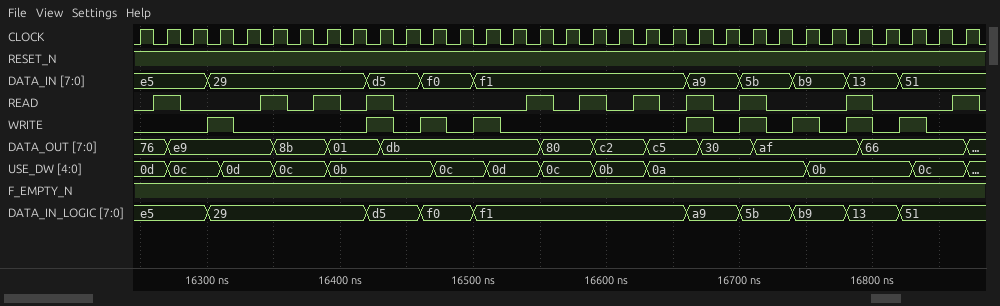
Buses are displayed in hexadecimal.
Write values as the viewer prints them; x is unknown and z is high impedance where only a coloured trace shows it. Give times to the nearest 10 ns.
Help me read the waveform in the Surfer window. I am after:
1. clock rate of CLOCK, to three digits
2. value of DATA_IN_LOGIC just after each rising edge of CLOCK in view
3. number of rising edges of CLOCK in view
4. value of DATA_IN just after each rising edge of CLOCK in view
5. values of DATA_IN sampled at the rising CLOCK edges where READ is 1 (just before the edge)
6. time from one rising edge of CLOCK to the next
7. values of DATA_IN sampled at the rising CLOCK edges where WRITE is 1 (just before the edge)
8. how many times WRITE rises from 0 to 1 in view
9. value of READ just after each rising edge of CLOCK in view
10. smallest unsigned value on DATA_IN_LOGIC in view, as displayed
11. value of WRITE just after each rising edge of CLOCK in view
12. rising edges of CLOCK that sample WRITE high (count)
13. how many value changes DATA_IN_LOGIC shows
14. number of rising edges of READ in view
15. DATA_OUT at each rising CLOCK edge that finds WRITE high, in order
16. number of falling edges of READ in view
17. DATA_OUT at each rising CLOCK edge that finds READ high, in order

50.0 MHz
e5, e5, e5, 29, 29, 29, 29, 29, 29, d5, d5, f0, f0, f1, f1, f1, f1, f1, f1, f1, f1, a9, a9, 5b, 5b, b9, b9, 13, 13, 51, 51, 51
32
e5, e5, e5, 29, 29, 29, 29, 29, 29, d5, d5, f0, f0, f1, f1, f1, f1, f1, f1, f1, f1, a9, a9, 5b, 5b, b9, b9, 13, 13, 51, 51, 51
e5, 29, 29, d5, f1, f1, f1, a9, 5b, 13, 51
20 ns
29, d5, f0, f1, a9, 5b, b9, 13, 51
9
0 1 0 0 0 1 0 1 0 1 0 0 0 0 0 1 0 1 0 1 0 1 0 1 0 0 0 1 0 0 0 1
13
0 0 0 1 0 0 0 0 0 1 0 1 0 1 0 0 0 0 0 0 0 1 0 1 0 1 0 1 0 1 0 0
9
9
11
e9, 01, db, db, c5, 30, af, af, 66
11
76, e9, 8b, 01, db, 80, c2, c5, 30, af, 66
